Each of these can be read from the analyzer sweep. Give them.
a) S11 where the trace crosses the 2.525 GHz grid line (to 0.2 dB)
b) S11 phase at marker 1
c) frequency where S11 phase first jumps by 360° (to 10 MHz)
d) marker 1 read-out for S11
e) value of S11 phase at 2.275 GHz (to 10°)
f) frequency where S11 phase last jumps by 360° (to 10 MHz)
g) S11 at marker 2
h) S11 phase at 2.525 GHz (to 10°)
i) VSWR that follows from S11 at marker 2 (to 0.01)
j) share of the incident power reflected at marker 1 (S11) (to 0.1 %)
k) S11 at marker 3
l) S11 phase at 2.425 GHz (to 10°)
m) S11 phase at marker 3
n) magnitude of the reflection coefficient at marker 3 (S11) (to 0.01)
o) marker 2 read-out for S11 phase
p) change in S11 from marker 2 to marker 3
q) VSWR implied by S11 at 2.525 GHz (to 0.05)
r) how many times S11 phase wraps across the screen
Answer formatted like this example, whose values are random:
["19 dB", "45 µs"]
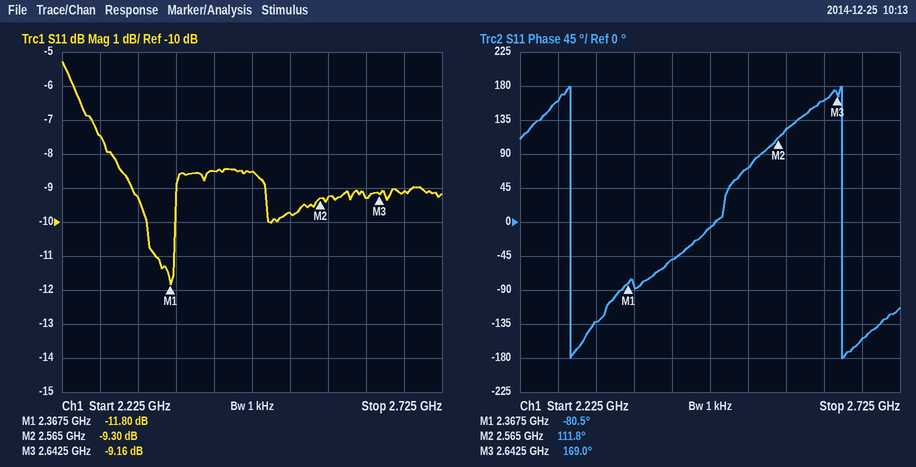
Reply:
["-9.8 dB", "-80.5°", "2.29 GHz", "-11.80 dB", "160°", "2.65 GHz", "-9.30 dB", "70°", "2.04", "6.6 %", "-9.16 dB", "-50°", "169.0°", "0.35", "111.8°", "0.14 dB", "1.95", "2"]
